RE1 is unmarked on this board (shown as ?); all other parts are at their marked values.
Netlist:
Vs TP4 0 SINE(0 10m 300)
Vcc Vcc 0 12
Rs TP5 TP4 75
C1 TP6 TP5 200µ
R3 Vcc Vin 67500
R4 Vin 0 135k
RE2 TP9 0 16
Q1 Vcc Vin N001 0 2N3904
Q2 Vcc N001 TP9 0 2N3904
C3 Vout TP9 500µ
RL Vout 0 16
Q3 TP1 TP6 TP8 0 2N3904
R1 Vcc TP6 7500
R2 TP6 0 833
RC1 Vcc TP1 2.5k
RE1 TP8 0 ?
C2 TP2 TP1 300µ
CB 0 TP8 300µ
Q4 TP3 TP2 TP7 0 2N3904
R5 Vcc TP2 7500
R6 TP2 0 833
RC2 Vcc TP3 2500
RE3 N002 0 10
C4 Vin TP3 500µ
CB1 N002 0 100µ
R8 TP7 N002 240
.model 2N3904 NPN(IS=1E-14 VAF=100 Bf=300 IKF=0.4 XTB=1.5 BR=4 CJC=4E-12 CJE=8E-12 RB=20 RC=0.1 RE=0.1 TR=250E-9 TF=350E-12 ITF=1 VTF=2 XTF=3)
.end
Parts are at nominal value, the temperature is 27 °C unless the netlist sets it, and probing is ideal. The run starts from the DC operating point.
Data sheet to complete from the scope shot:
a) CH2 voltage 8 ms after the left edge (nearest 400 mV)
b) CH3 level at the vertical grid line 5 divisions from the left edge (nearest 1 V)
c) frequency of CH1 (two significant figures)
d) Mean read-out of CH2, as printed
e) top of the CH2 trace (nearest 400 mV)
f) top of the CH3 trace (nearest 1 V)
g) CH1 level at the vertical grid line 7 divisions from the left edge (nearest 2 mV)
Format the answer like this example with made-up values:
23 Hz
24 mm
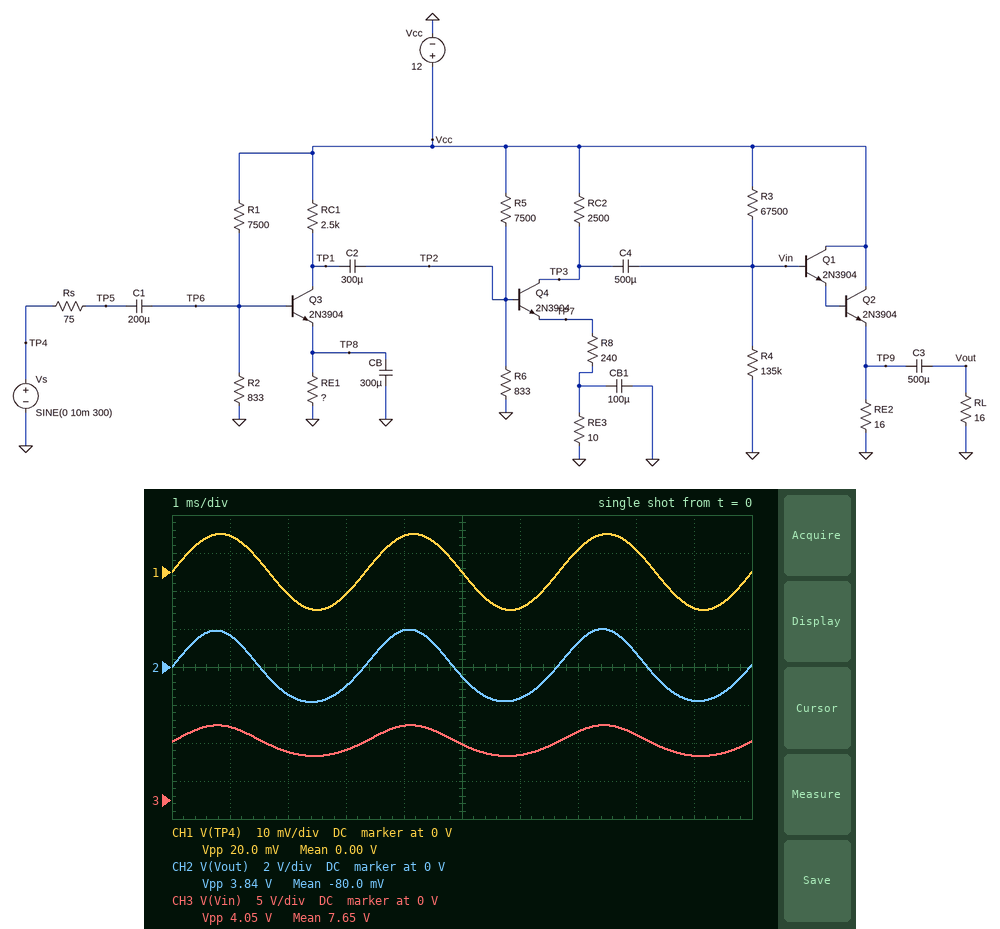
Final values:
800 mV
7 V
300 Hz
-80.0 mV
2.0 V
10 V
6 mV
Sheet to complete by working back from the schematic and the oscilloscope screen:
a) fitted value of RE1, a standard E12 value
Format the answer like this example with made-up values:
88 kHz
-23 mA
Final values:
470 Ω
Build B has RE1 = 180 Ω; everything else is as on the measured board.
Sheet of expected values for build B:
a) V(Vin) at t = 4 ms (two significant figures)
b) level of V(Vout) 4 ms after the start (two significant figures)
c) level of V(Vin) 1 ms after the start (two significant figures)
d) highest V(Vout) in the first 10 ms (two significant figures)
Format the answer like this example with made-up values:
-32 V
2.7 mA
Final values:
12 V
4.1 V
11 V
4.2 V
